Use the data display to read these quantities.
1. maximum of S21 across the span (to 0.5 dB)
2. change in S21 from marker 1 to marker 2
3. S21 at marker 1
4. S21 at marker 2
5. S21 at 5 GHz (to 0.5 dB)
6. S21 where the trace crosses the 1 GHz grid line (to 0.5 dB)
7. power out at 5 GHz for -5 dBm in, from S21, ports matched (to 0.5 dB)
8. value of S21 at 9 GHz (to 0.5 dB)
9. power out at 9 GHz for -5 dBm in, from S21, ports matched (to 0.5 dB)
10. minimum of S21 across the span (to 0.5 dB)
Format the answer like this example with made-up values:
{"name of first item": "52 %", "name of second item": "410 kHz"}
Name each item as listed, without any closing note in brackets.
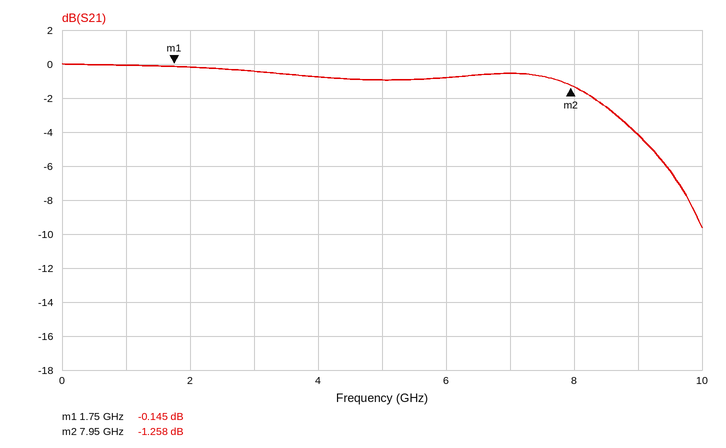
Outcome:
{"maximum of S21 across the span": "0.0 dB", "change in S21 from marker 1 to marker 2": "-1.113 dB", "S21 at marker 1": "-0.145 dB", "S21 at marker 2": "-1.258 dB", "S21 at 5 GHz": "-1.0 dB", "S21 where the trace crosses the 1 GHz grid line": "0.0 dB", "power out at 5 GHz for -5 dBm in, from S21, ports matched": "-6.0 dBm", "value of S21 at 9 GHz": "-4.0 dB", "power out at 9 GHz for -5 dBm in, from S21, ports matched": "-9.0 dBm", "minimum of S21 across the span": "-9.5 dB"}
